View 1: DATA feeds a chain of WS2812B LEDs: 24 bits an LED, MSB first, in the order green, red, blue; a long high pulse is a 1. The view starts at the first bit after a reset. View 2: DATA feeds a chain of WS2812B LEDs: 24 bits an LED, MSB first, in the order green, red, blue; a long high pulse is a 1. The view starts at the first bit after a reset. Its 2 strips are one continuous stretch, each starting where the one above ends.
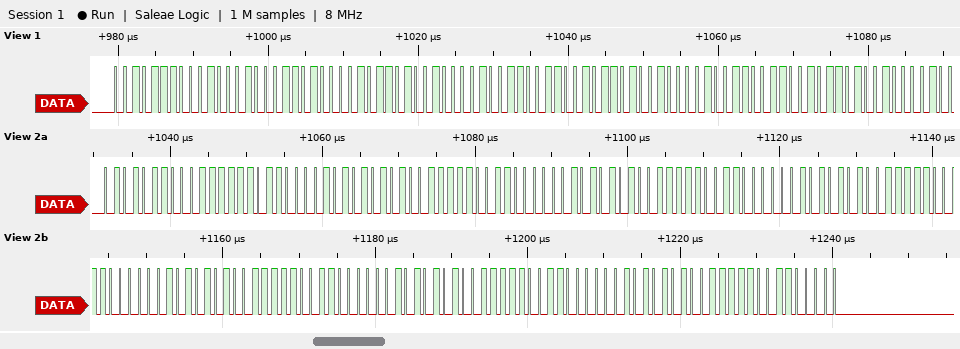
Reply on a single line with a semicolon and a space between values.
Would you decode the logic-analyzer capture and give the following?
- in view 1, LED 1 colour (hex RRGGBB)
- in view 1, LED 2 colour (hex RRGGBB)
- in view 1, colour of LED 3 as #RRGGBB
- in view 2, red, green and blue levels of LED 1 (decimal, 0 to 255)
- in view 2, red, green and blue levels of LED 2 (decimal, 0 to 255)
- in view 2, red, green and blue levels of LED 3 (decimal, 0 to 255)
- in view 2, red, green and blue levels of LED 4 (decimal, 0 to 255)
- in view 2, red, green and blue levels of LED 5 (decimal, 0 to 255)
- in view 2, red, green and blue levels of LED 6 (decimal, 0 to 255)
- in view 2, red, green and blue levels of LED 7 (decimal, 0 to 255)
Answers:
#222E34; #212D33; #212D33; 63, 86, 97; 62, 85, 96; 62, 85, 96; 62, 85, 96; 62, 85, 96; 62, 85, 96; 62, 85, 96
